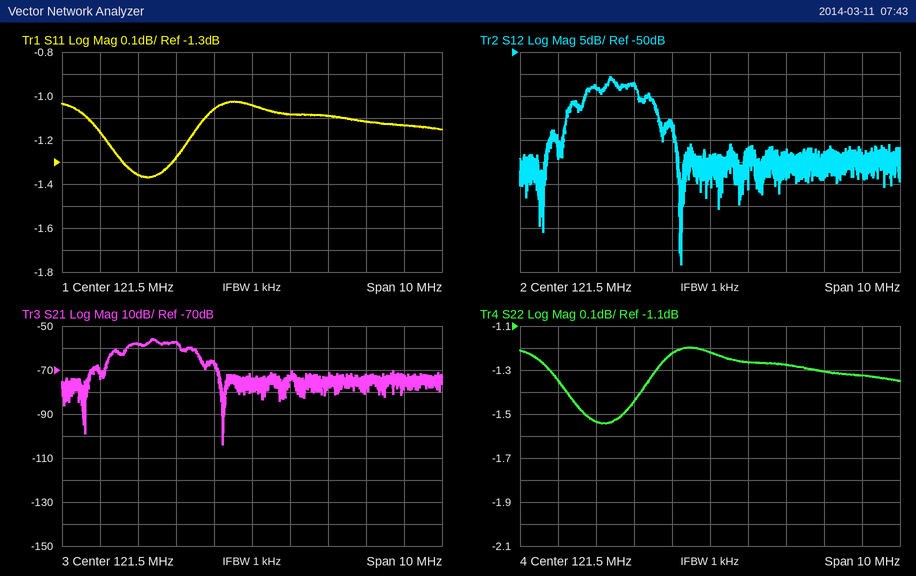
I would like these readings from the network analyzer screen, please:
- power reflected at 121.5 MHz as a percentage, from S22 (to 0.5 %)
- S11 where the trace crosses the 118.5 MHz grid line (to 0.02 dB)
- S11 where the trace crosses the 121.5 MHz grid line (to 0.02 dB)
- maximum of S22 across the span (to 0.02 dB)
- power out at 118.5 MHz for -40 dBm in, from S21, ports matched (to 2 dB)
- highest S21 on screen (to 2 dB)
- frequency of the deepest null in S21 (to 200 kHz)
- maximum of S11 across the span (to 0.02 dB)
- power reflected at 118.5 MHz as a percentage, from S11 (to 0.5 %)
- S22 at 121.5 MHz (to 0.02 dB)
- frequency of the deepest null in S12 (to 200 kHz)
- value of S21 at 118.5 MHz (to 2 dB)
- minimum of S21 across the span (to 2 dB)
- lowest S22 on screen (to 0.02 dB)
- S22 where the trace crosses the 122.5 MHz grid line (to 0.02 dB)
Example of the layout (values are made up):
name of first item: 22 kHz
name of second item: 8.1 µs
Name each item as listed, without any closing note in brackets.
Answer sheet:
power reflected at 121.5 MHz as a percentage, from S22: 75.5 %
S11 where the trace crosses the 118.5 MHz grid line: -1.36 dB
S11 where the trace crosses the 121.5 MHz grid line: -1.04 dB
maximum of S22 across the span: -1.20 dB
power out at 118.5 MHz for -40 dBm in, from S21, ports matched: -98 dBm
highest S21 on screen: -56 dB
frequency of the deepest null in S21: 120.8 MHz
maximum of S11 across the span: -1.02 dB
power reflected at 118.5 MHz as a percentage, from S11: 73.0 %
S22 at 121.5 MHz: -1.22 dB
frequency of the deepest null in S12: 120.8 MHz
value of S21 at 118.5 MHz: -58 dB
minimum of S21 across the span: -104 dB
lowest S22 on screen: -1.54 dB
S22 where the trace crosses the 122.5 MHz grid line: -1.26 dB
